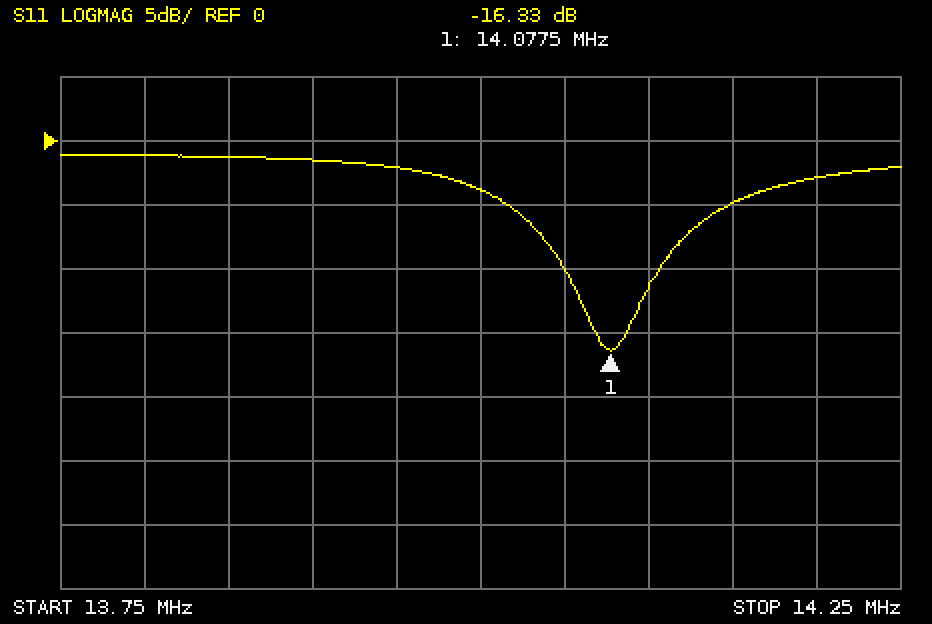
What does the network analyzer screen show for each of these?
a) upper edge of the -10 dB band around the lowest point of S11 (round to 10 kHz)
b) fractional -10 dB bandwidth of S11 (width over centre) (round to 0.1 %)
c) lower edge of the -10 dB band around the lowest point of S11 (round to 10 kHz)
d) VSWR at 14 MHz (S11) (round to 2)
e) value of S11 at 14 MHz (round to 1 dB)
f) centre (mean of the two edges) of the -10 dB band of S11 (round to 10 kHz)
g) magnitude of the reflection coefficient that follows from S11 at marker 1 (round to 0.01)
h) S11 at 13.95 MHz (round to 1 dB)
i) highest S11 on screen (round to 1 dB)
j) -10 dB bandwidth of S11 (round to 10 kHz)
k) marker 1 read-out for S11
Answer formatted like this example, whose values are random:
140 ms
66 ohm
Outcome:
14.11 MHz
0.4 %
14.05 MHz
4
-4 dB
14.08 MHz
0.15
-2 dB
-1 dB
60 kHz
-16.33 dB
